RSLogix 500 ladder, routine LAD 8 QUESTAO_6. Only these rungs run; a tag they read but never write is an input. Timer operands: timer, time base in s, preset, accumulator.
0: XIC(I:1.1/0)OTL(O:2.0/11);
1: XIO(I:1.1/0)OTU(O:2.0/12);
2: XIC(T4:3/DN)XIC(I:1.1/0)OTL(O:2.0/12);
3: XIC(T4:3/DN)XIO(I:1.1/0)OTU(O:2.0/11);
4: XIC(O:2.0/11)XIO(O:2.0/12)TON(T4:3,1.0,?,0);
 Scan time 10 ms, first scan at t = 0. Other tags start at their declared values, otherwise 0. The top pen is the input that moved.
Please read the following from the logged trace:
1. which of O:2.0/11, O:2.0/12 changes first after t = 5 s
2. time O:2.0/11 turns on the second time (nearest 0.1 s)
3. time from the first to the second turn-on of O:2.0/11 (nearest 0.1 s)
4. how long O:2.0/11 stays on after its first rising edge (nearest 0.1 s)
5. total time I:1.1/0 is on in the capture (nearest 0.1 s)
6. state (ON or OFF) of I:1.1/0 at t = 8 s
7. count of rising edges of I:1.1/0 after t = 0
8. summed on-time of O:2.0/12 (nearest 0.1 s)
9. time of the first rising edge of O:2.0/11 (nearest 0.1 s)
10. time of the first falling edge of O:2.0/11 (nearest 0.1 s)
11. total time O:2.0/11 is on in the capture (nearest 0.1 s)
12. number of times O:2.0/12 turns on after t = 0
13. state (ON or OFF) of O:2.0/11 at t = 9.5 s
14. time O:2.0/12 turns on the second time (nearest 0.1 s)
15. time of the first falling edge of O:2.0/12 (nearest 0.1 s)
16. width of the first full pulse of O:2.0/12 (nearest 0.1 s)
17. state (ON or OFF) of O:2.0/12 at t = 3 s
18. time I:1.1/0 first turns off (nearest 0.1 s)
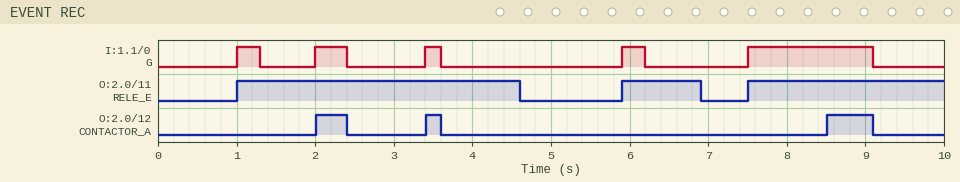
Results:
O:2.0/11
5.9 s
4.9 s
3.6 s
2.8 s
ON
5
1.2 s
1.0 s
4.6 s
7.1 s
3
ON
3.4 s
2.4 s
0.4 s
OFF
1.3 s
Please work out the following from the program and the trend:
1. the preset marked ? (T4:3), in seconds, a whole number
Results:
1 s
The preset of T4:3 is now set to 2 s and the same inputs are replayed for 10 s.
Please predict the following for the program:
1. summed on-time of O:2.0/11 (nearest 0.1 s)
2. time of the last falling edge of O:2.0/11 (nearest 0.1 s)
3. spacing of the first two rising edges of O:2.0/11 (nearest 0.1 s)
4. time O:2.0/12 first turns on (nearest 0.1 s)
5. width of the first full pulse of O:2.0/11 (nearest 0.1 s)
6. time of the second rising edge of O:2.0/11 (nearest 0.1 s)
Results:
8.1 s
5.4 s
2.4 s
7.9 s
2.0 s
3.4 s
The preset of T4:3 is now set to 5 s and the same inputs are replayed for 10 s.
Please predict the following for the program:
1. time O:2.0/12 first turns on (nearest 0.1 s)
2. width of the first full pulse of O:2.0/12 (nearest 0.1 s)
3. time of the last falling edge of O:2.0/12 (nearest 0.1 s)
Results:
6.0 s
0.2 s
6.2 s
